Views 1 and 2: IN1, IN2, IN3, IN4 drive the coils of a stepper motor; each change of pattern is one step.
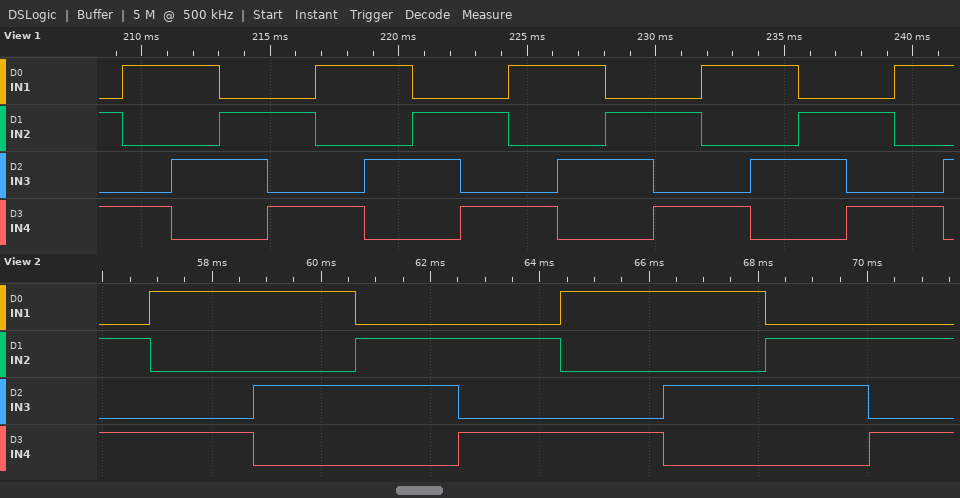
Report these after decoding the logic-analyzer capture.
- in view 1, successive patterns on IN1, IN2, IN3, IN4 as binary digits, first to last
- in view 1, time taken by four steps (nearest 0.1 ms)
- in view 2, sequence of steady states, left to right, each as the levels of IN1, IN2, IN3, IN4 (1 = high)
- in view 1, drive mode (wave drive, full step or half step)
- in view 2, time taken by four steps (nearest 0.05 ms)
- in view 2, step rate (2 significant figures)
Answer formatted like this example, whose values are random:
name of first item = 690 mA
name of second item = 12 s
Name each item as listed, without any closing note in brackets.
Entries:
in view 1, successive patterns on IN1, IN2, IN3, IN4 as binary digits, first to last = 0101 1001 1010 0110 0101 1001 1010 0110 0101 1001 1010 0110 0101 1001 1010 0110 0101 1001 1010
in view 1, time taken by four steps = 7.5 ms
in view 2, sequence of steady states, left to right, each as the levels of IN1, IN2, IN3, IN4 = 0101 1001 1010 0110 0101 1001 1010 0110 0101
in view 1, drive mode = full step
in view 2, time taken by four steps = 7.50 ms
in view 2, step rate = 530 steps/s
